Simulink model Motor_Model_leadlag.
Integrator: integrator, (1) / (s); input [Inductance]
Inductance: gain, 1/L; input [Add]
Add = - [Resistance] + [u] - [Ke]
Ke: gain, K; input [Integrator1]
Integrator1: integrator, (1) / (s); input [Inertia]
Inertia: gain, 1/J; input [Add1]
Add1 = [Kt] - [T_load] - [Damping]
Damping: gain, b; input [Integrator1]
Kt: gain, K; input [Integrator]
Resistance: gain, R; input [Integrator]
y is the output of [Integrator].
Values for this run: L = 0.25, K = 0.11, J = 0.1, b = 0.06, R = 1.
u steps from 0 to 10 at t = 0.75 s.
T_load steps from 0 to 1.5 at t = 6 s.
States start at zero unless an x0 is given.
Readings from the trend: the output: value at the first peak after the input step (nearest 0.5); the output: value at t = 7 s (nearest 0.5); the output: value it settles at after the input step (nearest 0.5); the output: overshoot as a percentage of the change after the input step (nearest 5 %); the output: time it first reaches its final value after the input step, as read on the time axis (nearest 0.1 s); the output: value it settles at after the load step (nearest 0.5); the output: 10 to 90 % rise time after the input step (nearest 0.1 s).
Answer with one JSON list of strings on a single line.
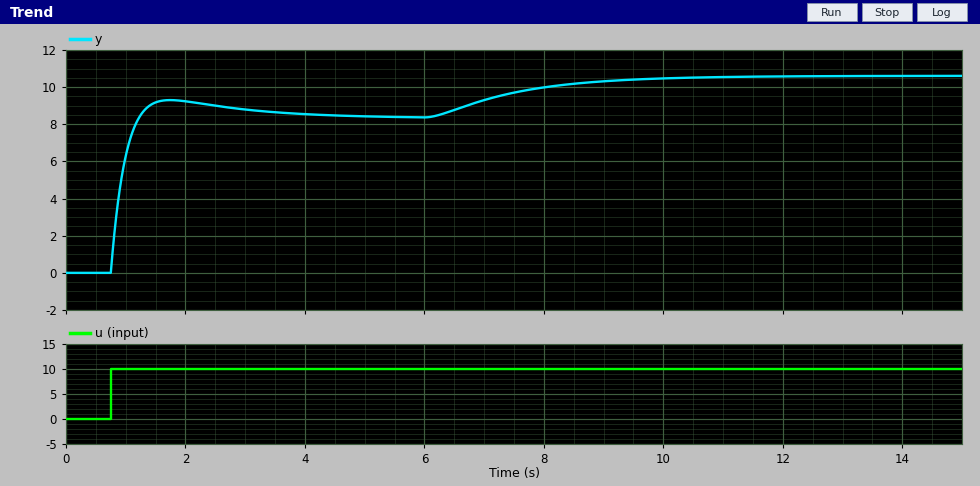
["9.5", "9.5", "8.5", "10 %", "1.2 s", "10.5", "0.3 s"]
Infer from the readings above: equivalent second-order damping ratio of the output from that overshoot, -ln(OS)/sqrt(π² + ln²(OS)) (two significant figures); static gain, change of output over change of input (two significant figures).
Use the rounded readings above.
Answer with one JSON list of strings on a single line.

["0.59", "0.85"]
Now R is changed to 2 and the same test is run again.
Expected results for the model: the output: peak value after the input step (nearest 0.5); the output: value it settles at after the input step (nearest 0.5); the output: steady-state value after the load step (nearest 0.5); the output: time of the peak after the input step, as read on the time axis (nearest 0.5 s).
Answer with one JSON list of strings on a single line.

["5.0", "4.5", "6.0", "1.5 s"]
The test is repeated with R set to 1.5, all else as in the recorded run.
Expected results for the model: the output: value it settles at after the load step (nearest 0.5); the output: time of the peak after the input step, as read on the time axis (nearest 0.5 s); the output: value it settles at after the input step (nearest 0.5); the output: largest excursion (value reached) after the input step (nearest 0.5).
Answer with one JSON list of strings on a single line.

["7.5", "1.5 s", "6.0", "6.5"]
